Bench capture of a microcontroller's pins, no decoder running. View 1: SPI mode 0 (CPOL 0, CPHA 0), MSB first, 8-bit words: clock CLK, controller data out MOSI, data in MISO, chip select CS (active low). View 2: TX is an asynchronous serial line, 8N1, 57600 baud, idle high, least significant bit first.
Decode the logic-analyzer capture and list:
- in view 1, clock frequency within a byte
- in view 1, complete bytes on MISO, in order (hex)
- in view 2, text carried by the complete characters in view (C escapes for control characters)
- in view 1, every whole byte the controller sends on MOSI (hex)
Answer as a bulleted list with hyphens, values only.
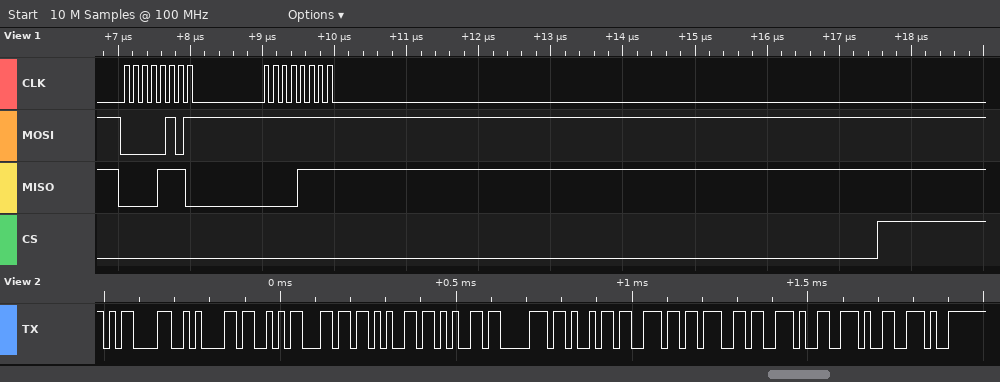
- 8 MHz
- 0E 0F
- "\r\nSleeping..."
- 05 FF
